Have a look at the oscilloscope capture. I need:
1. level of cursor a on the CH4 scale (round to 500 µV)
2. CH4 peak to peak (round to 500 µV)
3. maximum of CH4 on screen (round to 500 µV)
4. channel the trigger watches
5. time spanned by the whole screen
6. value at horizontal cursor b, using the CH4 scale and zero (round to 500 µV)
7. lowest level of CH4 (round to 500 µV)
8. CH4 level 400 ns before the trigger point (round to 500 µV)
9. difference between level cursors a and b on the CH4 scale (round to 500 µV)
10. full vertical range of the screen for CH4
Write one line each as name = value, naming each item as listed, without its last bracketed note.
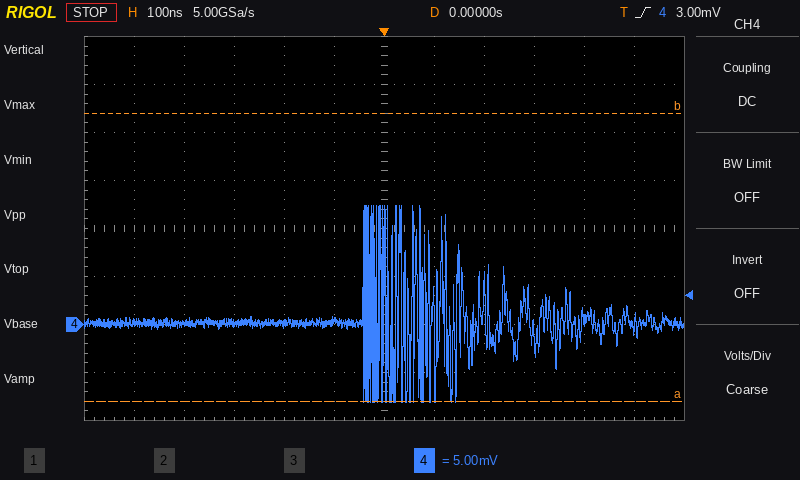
level of cursor a on the CH4 scale = -8.0 mV
CH4 peak to peak = 20.5 mV
maximum of CH4 on screen = 12.5 mV
channel the trigger watches = CH4
time spanned by the whole screen = 1.2 µs
value at horizontal cursor b, using the CH4 scale and zero = 22.0 mV
lowest level of CH4 = -8.0 mV
CH4 level 400 ns before the trigger point = 0.0 mV
difference between level cursors a and b on the CH4 scale = 30.0 mV
full vertical range of the screen for CH4 = 40 mV
